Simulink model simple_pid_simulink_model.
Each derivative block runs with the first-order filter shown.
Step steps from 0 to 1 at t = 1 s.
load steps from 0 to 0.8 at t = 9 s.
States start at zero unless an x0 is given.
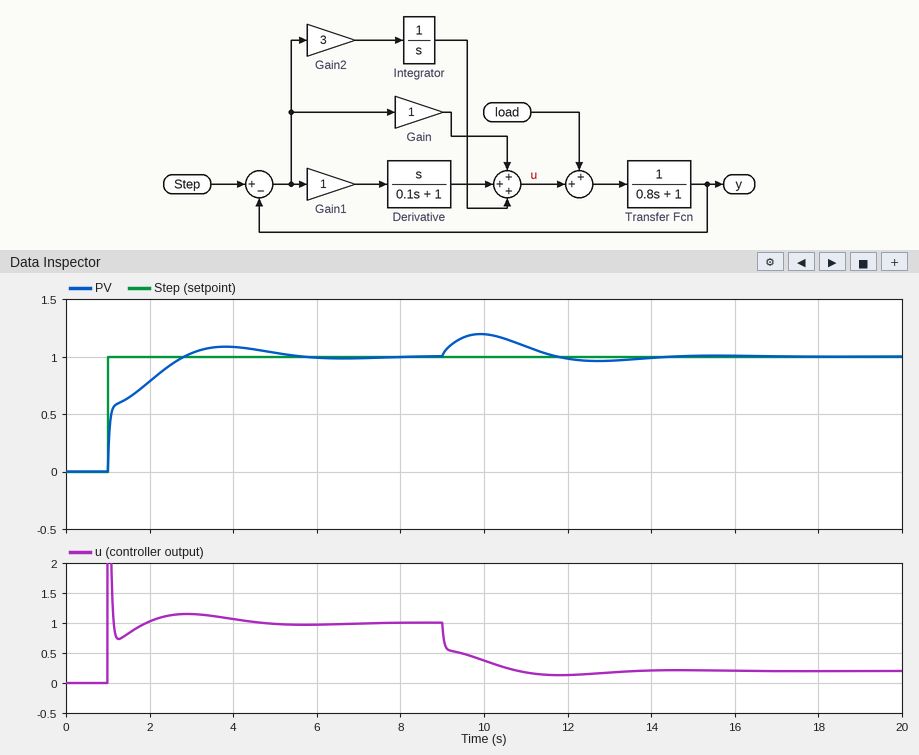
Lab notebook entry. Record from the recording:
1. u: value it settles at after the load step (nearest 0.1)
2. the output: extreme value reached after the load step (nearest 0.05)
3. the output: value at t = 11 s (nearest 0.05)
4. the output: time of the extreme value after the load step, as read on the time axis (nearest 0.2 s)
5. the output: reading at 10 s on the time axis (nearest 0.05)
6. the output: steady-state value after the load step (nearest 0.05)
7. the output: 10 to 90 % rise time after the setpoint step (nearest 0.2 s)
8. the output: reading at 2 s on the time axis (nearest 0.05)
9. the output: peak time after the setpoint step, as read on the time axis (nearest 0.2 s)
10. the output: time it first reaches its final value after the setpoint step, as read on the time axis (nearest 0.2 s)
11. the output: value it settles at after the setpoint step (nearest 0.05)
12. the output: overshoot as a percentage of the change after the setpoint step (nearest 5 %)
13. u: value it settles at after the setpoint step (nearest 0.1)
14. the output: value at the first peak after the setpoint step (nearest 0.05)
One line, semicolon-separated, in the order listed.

0.2; 1.20; 1.10; 10.0 s; 1.20; 1.00; 1.4 s; 0.80; 3.8 s; 2.8 s; 1.00; 10 %; 1.0; 1.10
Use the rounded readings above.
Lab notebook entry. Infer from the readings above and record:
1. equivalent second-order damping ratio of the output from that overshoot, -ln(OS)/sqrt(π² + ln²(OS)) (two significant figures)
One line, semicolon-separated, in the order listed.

0.59
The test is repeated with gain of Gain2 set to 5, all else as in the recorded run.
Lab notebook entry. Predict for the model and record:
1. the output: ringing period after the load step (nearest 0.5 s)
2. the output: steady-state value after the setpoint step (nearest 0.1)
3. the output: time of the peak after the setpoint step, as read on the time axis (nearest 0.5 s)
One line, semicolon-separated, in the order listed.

4.0 s; 1.0; 3.0 s
